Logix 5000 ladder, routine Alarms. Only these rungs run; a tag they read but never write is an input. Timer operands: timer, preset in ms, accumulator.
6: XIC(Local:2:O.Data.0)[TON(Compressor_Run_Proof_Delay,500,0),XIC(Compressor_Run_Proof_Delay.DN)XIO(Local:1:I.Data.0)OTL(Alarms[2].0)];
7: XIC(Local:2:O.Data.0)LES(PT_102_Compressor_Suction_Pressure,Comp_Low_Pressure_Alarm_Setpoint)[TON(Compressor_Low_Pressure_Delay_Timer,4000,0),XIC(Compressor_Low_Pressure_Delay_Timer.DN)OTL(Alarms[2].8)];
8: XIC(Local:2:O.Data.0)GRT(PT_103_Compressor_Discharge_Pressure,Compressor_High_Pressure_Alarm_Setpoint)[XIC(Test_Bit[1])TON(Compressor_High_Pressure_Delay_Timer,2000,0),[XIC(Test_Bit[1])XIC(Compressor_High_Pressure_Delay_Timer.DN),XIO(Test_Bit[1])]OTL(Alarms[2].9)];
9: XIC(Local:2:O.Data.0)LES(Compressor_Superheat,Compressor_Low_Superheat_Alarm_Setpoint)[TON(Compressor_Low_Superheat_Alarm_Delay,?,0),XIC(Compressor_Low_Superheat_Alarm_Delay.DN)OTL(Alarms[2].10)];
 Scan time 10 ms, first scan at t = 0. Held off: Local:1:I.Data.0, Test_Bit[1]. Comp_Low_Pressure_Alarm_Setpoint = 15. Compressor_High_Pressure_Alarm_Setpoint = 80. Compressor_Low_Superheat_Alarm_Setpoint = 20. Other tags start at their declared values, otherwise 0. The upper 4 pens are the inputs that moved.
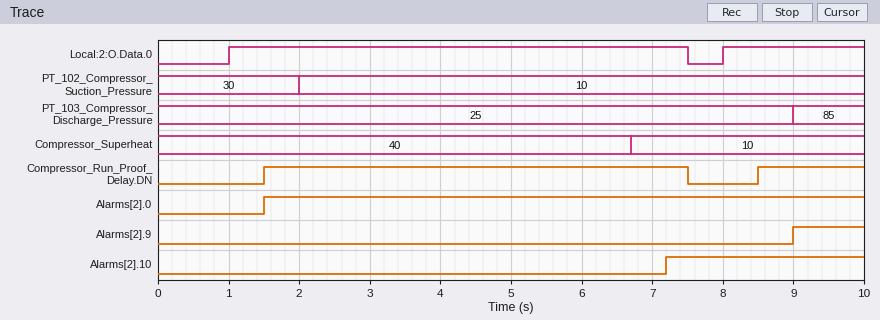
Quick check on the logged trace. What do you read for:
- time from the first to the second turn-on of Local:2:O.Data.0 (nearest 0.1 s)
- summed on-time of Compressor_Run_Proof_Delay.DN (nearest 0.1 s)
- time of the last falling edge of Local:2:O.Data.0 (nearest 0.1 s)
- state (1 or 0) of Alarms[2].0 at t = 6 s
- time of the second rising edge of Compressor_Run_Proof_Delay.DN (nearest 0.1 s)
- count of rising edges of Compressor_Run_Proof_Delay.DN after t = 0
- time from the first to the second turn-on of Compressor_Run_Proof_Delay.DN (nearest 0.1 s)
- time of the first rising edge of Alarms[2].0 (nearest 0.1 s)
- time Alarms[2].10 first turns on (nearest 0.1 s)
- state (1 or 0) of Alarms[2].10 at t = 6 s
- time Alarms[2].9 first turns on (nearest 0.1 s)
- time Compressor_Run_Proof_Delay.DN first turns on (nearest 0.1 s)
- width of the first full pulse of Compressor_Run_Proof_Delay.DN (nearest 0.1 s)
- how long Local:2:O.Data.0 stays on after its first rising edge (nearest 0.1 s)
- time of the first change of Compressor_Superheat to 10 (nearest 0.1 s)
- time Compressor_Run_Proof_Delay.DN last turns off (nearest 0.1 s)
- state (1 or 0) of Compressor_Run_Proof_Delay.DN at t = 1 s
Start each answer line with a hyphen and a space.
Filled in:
- 7.0 s
- 7.5 s
- 7.5 s
- 1
- 8.5 s
- 2
- 7.0 s
- 1.5 s
- 7.2 s
- 0
- 9.0 s
- 1.5 s
- 6.0 s
- 6.5 s
- 6.7 s
- 7.5 s
- 0
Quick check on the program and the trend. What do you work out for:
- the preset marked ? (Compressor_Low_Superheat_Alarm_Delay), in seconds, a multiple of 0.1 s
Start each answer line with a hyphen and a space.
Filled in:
- 0.5 s
